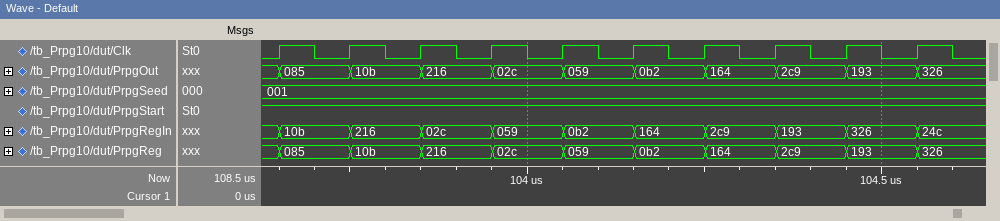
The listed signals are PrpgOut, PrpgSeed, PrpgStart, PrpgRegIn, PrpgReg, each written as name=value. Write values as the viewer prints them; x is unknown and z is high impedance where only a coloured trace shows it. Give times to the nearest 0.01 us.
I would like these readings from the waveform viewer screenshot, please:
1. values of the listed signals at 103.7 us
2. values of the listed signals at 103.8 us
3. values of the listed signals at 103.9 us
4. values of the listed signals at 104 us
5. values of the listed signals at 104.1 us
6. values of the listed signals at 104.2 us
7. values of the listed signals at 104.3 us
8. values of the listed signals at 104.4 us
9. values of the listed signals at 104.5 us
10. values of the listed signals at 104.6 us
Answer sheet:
PrpgOut=085, PrpgSeed=001, PrpgStart=1, PrpgRegIn=10b, PrpgReg=085
PrpgOut=10b, PrpgSeed=001, PrpgStart=1, PrpgRegIn=216, PrpgReg=10b
PrpgOut=216, PrpgSeed=001, PrpgStart=1, PrpgRegIn=02c, PrpgReg=216
PrpgOut=02c, PrpgSeed=001, PrpgStart=1, PrpgRegIn=059, PrpgReg=02c
PrpgOut=059, PrpgSeed=001, PrpgStart=1, PrpgRegIn=0b2, PrpgReg=059
PrpgOut=0b2, PrpgSeed=001, PrpgStart=1, PrpgRegIn=164, PrpgReg=0b2
PrpgOut=164, PrpgSeed=001, PrpgStart=1, PrpgRegIn=2c9, PrpgReg=164
PrpgOut=2c9, PrpgSeed=001, PrpgStart=1, PrpgRegIn=193, PrpgReg=2c9
PrpgOut=193, PrpgSeed=001, PrpgStart=1, PrpgRegIn=326, PrpgReg=193
PrpgOut=326, PrpgSeed=001, PrpgStart=1, PrpgRegIn=24c, PrpgReg=326
